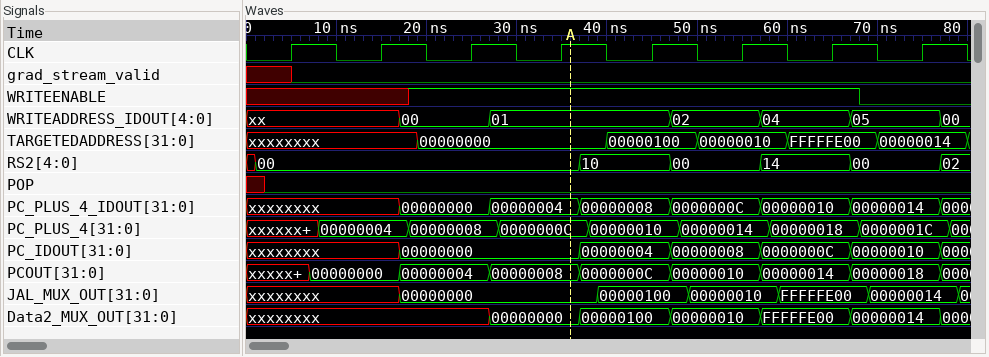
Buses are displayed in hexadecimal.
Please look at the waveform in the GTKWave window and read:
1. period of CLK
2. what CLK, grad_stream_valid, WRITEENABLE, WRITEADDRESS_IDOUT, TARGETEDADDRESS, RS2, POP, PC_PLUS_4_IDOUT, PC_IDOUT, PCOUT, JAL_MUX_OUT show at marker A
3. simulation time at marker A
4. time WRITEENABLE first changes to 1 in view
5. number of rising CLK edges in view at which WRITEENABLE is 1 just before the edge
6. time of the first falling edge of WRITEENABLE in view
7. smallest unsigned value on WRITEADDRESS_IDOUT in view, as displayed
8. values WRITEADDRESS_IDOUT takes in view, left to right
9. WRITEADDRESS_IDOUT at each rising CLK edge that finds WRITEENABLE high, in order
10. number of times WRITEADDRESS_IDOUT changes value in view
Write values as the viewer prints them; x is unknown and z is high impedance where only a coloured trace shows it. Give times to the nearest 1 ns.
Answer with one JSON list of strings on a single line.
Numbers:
["10 ns", "CLK=1, grad_stream_valid=0, WRITEENABLE=1, WRITEADDRESS_IDOUT=01, TARGETEDADDRESS=00000000, RS2=00, POP=0, PC_PLUS_4_IDOUT=00000004, PC_IDOUT=00000000, PCOUT=00000008, JAL_MUX_OUT=00000000", "36 ns", "18 ns", "5", "68 ns", "00", "xx, 00, 01, 02, 04, 05, 00", "00, 01, 01, 02, 04", "6"]
